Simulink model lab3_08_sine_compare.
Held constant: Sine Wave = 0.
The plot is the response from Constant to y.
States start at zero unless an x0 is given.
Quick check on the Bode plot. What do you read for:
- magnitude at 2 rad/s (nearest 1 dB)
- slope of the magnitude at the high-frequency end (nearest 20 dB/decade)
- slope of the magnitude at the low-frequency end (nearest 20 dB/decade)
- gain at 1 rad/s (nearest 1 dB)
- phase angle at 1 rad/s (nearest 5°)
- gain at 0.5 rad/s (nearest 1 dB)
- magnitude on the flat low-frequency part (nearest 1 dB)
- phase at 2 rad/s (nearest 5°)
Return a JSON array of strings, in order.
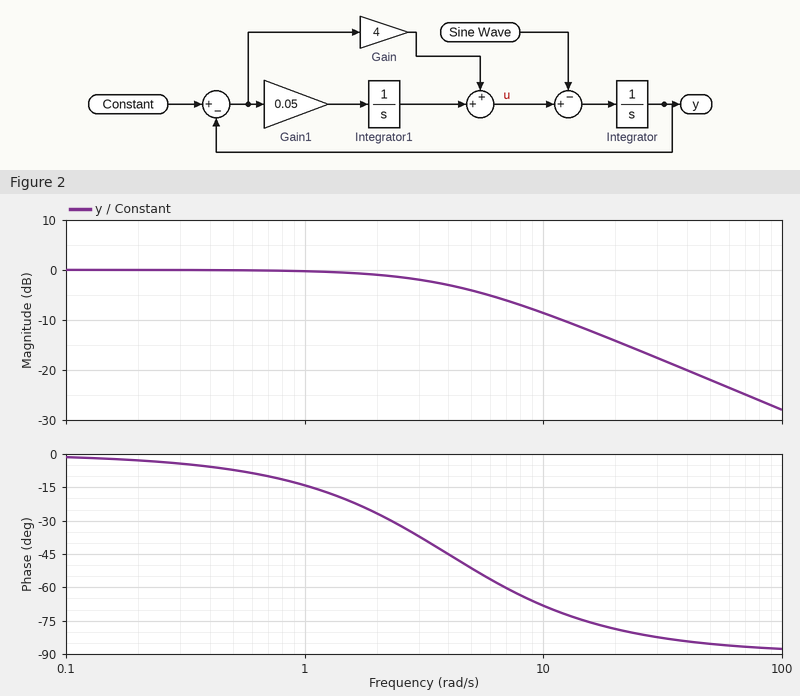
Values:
["-1 dB", "-20 dB/decade", "0 dB/decade", "0 dB", "-15°", "0 dB", "0 dB", "-25°"]
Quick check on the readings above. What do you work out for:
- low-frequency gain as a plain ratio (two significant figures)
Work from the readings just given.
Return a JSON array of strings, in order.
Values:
["1.0"]
